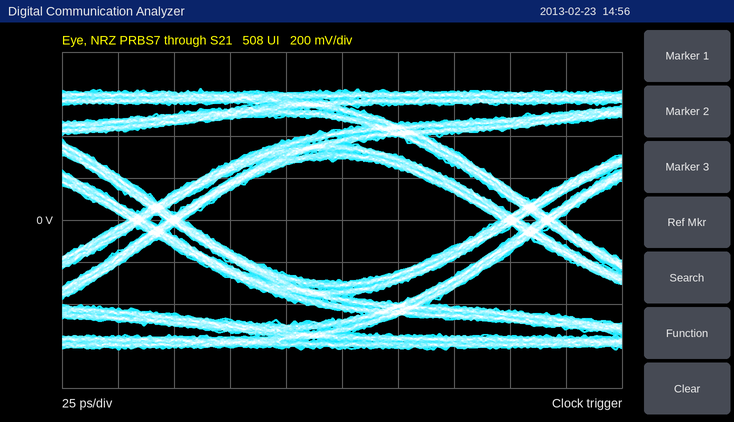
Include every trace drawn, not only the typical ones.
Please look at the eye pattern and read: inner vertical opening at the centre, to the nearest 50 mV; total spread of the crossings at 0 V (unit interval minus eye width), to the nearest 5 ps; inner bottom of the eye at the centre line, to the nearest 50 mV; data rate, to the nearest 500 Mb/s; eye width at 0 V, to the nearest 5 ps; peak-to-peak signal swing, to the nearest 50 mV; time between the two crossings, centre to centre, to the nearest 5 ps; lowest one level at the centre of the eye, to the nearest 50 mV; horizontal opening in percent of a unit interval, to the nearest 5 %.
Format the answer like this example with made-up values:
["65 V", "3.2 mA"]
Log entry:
["600 mV", "25 ps", "-300 mV", "6.0 Gb/s", "140 ps", "1.25 V", "165 ps", "300 mV", "85 %"]
